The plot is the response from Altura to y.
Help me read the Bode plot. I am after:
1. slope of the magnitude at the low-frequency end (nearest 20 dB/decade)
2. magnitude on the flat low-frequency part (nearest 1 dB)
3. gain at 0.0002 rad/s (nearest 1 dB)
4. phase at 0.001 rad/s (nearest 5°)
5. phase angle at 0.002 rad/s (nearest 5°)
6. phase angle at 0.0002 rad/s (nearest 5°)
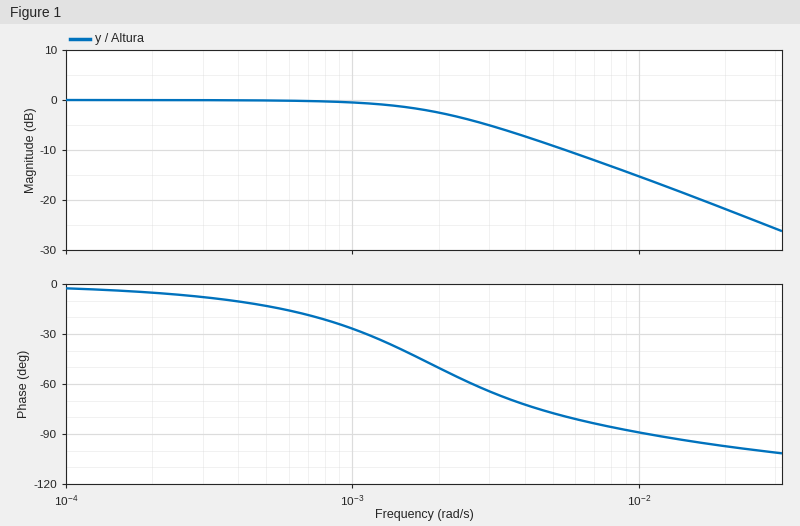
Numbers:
0 dB/decade
0 dB
0 dB
-25°
-50°
-5°
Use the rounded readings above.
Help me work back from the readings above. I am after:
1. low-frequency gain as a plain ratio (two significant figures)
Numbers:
1.0
